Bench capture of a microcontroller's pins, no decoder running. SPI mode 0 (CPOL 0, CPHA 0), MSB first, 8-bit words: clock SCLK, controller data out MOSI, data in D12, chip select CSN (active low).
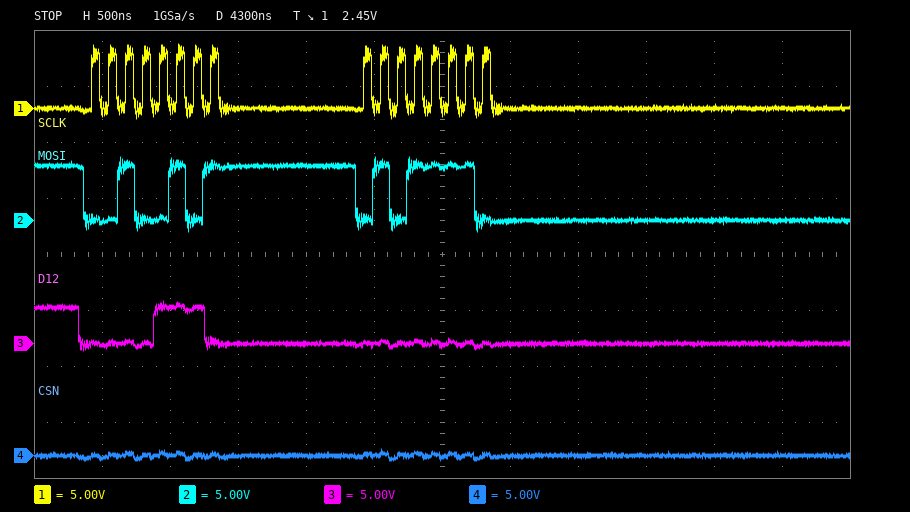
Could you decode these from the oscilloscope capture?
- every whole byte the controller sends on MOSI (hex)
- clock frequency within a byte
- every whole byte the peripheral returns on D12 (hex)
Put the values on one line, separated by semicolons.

25 5E; 8 MHz; 0E 00
